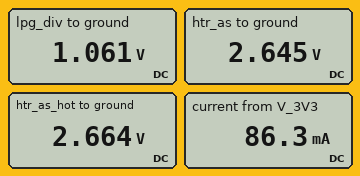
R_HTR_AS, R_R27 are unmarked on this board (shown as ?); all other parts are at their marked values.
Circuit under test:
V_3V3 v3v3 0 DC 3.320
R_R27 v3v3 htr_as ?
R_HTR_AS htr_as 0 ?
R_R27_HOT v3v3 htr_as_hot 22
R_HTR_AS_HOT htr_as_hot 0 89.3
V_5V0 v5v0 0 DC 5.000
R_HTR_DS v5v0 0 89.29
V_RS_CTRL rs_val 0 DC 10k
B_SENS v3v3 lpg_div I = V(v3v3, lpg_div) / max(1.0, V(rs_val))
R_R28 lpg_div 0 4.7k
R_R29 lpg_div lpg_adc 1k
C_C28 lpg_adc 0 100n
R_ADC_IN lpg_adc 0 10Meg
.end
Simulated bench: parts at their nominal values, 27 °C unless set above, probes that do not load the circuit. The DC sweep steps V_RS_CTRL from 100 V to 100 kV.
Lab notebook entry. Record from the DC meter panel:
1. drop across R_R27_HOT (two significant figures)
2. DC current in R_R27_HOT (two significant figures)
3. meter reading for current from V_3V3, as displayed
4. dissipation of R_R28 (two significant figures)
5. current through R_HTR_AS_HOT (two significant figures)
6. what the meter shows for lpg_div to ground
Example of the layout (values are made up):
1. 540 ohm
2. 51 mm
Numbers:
1. 660 mV
2. 30 mA
3. 86.3 mA
4. 240 µW
5. 30 mA
6. 1.061 V
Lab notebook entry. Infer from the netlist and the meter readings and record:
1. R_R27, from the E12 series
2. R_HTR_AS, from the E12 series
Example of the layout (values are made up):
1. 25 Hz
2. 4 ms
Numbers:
1. 12 Ω
2. 47 Ω
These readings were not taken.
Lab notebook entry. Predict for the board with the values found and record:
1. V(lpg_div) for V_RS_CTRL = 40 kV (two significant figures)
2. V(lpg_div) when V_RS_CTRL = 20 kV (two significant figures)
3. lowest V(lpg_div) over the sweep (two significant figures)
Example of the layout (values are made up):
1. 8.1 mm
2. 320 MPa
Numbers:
1. 350 mV
2. 630 mV
3. 150 mV
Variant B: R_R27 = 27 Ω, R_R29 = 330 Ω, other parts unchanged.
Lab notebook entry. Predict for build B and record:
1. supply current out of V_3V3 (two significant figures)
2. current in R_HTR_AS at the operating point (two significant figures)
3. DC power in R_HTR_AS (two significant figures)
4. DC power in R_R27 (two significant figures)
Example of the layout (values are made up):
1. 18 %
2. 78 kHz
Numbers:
1. 75 mA
2. 45 mA
3. 95 mW
4. 54 mW
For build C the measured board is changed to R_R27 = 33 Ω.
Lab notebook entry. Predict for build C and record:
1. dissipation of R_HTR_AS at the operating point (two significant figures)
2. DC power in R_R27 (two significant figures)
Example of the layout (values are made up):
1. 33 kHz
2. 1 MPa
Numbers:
1. 81 mW
2. 57 mW
